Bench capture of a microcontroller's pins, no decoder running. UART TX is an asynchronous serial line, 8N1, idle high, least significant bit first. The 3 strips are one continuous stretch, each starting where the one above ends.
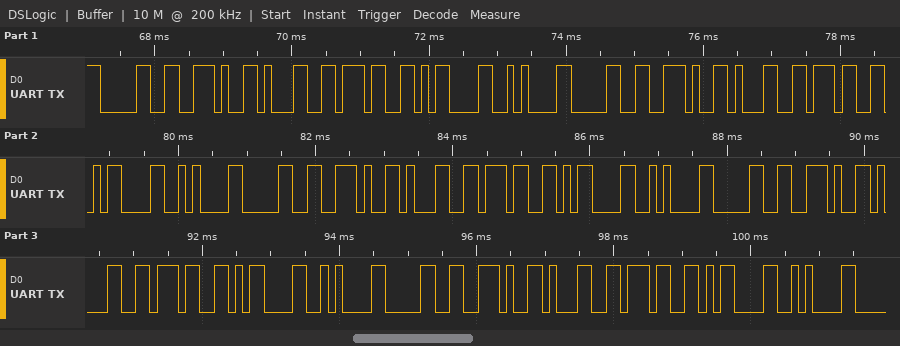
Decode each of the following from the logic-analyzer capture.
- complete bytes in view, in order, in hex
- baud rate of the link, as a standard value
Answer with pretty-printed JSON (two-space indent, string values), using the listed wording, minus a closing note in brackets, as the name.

{
  "complete bytes in view, in order, in hex": "30 2E 31 37 0D 0A 30 2E 31 37 0D 0A 30 2E 31 37 0D 0A 30 2E 31 37 0D 0A 30 2E 31 37 0D 0A",
  "baud rate of the link, as a standard value": "9600 baud"
}
